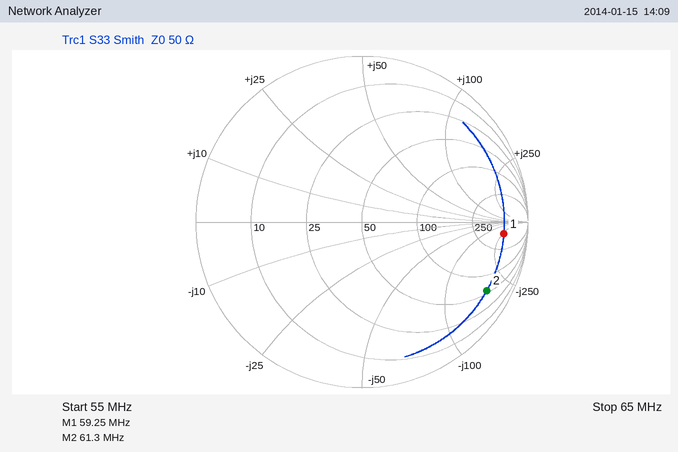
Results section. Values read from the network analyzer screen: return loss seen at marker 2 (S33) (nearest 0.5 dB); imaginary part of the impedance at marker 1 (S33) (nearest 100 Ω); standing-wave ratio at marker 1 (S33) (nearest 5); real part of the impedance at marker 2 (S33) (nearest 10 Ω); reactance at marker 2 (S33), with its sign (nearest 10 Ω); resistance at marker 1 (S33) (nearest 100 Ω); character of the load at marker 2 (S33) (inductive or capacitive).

1.5 dB
-300 Ω
15
60 Ω
-180 Ω
500 Ω
capacitive
